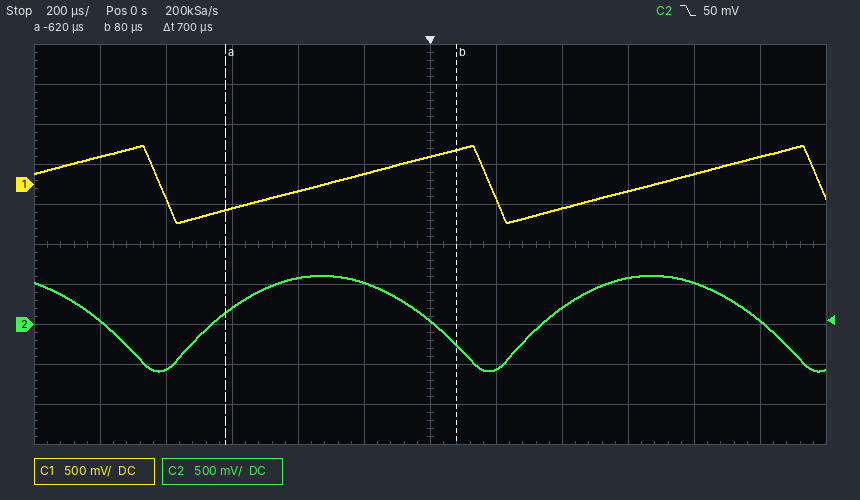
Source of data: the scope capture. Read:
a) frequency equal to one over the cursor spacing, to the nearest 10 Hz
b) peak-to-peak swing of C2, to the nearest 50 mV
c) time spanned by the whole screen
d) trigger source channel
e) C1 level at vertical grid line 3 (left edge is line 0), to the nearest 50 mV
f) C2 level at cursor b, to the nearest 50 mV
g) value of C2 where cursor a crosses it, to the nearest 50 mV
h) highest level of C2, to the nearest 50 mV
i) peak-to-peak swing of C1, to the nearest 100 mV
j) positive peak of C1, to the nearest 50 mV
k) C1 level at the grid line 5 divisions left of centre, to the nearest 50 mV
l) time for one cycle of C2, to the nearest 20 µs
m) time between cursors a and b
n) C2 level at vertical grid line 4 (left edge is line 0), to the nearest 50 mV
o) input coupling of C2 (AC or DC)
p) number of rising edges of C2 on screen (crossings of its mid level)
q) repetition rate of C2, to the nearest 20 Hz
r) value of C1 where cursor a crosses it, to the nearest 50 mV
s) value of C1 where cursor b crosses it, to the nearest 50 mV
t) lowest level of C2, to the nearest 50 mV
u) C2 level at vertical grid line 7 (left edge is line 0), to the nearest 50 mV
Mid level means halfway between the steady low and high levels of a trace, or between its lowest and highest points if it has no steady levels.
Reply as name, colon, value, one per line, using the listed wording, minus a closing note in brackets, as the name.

frequency equal to one over the cursor spacing, to the nearest 10 Hz: 1.43 kHz
peak-to-peak swing of C2, to the nearest 50 mV: 1.20 V
time spanned by the whole screen: 2.4 ms
trigger source channel: C2
C1 level at vertical grid line 3 (left edge is line 0), to the nearest 50 mV: -300 mV
C2 level at cursor b, to the nearest 50 mV: -250 mV
value of C2 where cursor a crosses it, to the nearest 50 mV: 150 mV
highest level of C2, to the nearest 50 mV: 600 mV
peak-to-peak swing of C1, to the nearest 100 mV: 1.00 V
positive peak of C1, to the nearest 50 mV: 500 mV
C1 level at the grid line 5 divisions left of centre, to the nearest 50 mV: 350 mV
time for one cycle of C2, to the nearest 20 µs: 1.00 ms
time between cursors a and b: 700 µs
C2 level at vertical grid line 4 (left edge is line 0), to the nearest 50 mV: 600 mV
input coupling of C2: DC
number of rising edges of C2 on screen: 2
repetition rate of C2, to the nearest 20 Hz: 1.00 kHz
value of C1 where cursor a crosses it, to the nearest 50 mV: -300 mV
value of C1 where cursor b crosses it, to the nearest 50 mV: 450 mV
lowest level of C2, to the nearest 50 mV: -600 mV
C2 level at vertical grid line 7 (left edge is line 0), to the nearest 50 mV: -550 mV
